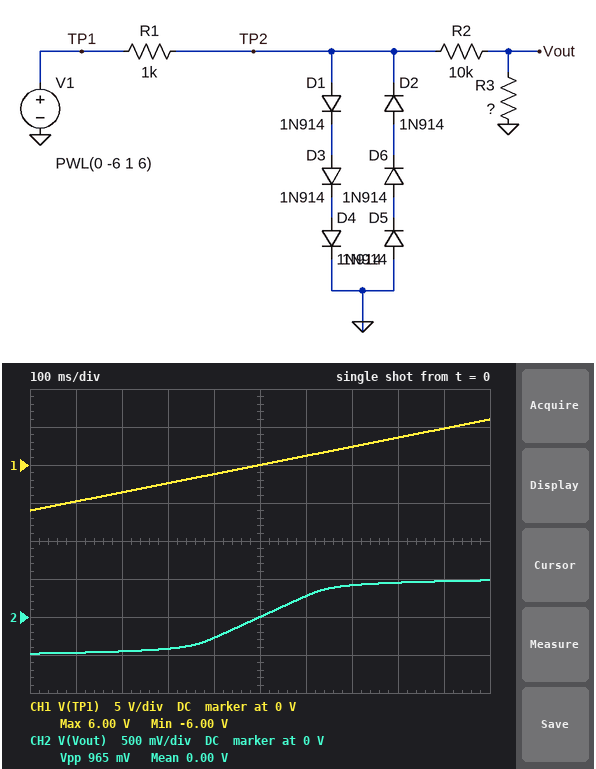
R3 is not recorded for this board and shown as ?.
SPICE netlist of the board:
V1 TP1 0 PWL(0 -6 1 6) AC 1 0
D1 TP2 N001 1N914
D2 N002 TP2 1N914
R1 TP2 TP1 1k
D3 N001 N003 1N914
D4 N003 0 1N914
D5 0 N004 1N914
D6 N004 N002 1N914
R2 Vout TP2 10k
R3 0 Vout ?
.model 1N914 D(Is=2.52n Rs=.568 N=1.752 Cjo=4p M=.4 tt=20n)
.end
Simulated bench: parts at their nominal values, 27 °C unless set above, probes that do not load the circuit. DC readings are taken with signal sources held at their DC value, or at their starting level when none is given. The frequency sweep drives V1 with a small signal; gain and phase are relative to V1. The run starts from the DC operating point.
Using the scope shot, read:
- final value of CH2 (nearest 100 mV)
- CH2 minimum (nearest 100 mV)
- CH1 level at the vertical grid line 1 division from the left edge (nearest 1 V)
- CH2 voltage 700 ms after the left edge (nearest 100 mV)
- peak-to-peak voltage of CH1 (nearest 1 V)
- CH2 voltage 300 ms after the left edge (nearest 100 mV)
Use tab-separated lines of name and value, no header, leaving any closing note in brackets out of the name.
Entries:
final value of CH2	500 mV
CH2 minimum	-500 mV
CH1 level at the vertical grid line 1 division from the left edge	-5 V
CH2 voltage 700 ms after the left edge	400 mV
peak-to-peak voltage of CH1	12 V
CH2 voltage 300 ms after the left edge	-400 mV
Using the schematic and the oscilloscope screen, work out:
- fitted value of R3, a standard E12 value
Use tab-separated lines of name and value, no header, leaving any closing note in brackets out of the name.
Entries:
fitted value of R3, a standard E12 value	3.3 kΩ
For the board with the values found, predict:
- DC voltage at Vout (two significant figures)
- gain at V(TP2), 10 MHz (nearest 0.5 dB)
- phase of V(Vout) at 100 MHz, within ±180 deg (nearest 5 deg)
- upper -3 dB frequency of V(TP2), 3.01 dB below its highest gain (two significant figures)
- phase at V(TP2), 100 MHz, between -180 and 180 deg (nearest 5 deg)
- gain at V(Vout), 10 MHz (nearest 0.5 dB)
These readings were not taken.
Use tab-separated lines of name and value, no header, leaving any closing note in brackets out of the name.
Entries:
DC voltage at Vout	-480 mV
gain at V(TP2), 10 MHz	-33.0 dB
phase of V(Vout) at 100 MHz, within ±180 deg	-55 deg
upper -3 dB frequency of V(TP2), 3.01 dB below its highest gain	8.2 MHz
phase at V(TP2), 100 MHz, between -180 and 180 deg	-55 deg
gain at V(Vout), 10 MHz	-45.0 dB
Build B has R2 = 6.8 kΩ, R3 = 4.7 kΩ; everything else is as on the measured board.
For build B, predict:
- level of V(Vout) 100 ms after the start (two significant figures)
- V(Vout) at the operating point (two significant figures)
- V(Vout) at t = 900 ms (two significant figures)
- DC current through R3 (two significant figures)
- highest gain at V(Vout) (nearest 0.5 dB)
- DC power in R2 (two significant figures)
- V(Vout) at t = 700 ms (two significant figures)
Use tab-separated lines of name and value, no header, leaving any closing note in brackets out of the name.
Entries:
level of V(Vout) 100 ms after the start	-770 mV
V(Vout) at the operating point	-790 mV
V(Vout) at t = 900 ms	770 mV
DC current through R3	170 µA
highest gain at V(Vout)	-37.0 dB
DC power in R2	190 µW
V(Vout) at t = 700 ms	690 mV
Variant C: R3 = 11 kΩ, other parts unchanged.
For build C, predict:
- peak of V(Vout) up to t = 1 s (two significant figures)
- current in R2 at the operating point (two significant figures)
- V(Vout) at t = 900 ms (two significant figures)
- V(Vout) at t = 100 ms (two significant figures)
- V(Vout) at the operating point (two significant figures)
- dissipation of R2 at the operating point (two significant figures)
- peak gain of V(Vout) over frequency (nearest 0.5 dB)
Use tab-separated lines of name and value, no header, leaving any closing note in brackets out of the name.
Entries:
peak of V(Vout) up to t = 1 s	1.0 V
current in R2 at the operating point	93 µA
V(Vout) at t = 900 ms	990 mV
V(Vout) at t = 100 ms	-990 mV
V(Vout) at the operating point	-1.0 V
dissipation of R2 at the operating point	86 µW
peak gain of V(Vout) over frequency	-35.0 dB
